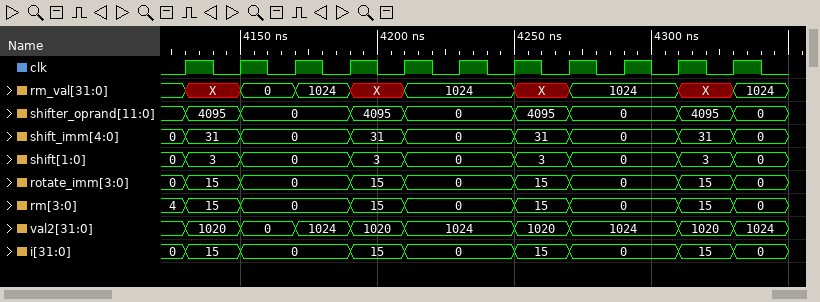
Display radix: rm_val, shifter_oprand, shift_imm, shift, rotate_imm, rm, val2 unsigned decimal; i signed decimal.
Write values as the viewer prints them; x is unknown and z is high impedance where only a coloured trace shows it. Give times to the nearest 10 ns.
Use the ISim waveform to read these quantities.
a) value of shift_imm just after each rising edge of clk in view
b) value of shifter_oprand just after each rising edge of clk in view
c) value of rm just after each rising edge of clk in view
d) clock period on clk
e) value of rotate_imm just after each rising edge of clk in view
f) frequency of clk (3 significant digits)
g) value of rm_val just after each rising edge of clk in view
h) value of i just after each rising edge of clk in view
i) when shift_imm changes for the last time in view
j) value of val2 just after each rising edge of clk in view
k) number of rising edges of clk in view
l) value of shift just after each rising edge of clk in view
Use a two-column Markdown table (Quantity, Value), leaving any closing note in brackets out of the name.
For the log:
| Quantity | Value |
|---|---|
| value of shift_imm just after each rising edge of clk in view | 31, 0, 0, 31, 0, 0, 31, 0, 0, 31, 0 |
| value of shifter_oprand just after each rising edge of clk in view | 4095, 0, 0, 4095, 0, 0, 4095, 0, 0, 4095, 0 |
| value of rm just after each rising edge of clk in view | 15, 0, 0, 15, 0, 0, 15, 0, 0, 15, 0 |
| clock period on clk | 20 ns |
| value of rotate_imm just after each rising edge of clk in view | 15, 0, 0, 15, 0, 0, 15, 0, 0, 15, 0 |
| frequency of clk | 50.0 MHz |
| value of rm_val just after each rising edge of clk in view | X, 0, 1024, X, 1024, 1024, X, 1024, 1024, X, 1024 |
| value of i just after each rising edge of clk in view | 15, 0, 0, 15, 0, 0, 15, 0, 0, 15, 0 |
| when shift_imm changes for the last time in view | 4330 ns |
| value of val2 just after each rising edge of clk in view | 1020, 0, 1024, 1020, 1024, 1024, 1020, 1024, 1024, 1020, 1024 |
| number of rising edges of clk in view | 11 |
| value of shift just after each rising edge of clk in view | 3, 0, 0, 3, 0, 0, 3, 0, 0, 3, 0 |
